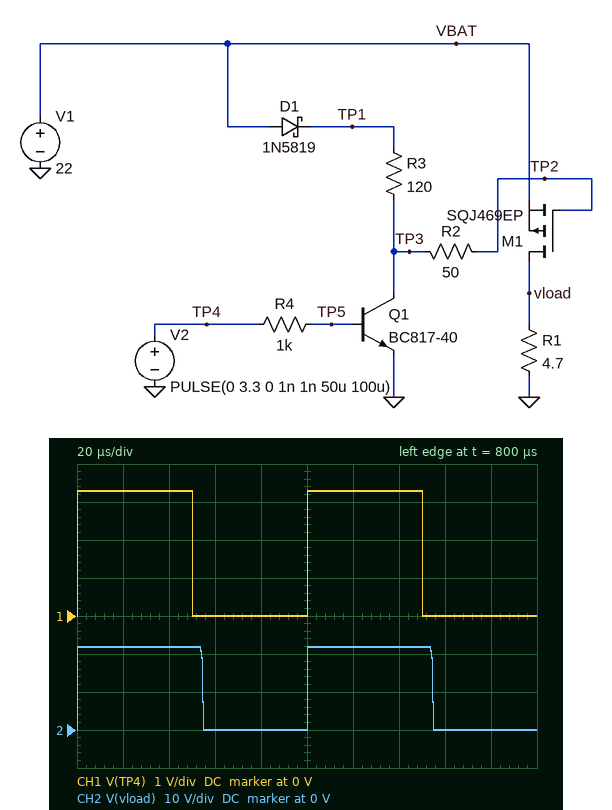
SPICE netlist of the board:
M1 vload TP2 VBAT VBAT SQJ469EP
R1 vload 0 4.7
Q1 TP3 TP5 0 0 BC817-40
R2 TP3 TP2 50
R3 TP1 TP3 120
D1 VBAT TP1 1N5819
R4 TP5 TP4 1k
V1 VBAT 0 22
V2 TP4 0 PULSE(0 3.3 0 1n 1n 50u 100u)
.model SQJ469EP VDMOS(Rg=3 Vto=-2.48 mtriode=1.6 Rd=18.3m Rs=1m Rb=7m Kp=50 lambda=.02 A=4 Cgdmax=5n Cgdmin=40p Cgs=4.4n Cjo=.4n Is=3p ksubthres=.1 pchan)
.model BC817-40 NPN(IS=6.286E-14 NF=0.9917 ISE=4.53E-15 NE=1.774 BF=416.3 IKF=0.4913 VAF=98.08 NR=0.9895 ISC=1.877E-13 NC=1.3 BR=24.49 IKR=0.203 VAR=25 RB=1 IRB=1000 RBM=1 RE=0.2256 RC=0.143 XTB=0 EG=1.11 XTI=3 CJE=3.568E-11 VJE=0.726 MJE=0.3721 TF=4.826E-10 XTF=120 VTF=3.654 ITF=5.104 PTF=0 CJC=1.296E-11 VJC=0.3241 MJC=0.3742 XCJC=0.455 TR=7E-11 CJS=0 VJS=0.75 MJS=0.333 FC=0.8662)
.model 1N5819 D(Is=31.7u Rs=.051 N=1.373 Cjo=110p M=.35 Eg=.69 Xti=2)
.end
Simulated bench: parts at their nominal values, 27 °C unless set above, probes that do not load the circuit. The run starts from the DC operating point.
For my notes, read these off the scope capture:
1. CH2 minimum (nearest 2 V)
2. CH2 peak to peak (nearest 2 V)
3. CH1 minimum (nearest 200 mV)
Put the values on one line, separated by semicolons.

0 V; 22 V; 0 V
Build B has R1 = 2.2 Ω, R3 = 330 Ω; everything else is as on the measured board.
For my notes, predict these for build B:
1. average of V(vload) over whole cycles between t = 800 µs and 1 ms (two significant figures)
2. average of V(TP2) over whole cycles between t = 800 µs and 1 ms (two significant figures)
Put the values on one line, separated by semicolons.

13 V; 10 V
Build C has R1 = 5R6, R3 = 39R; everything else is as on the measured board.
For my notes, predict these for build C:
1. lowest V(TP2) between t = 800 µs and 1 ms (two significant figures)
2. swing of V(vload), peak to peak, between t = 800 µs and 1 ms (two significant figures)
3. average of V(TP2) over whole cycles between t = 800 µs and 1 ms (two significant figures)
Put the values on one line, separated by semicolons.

2.5 V; 22 V; 12 V
